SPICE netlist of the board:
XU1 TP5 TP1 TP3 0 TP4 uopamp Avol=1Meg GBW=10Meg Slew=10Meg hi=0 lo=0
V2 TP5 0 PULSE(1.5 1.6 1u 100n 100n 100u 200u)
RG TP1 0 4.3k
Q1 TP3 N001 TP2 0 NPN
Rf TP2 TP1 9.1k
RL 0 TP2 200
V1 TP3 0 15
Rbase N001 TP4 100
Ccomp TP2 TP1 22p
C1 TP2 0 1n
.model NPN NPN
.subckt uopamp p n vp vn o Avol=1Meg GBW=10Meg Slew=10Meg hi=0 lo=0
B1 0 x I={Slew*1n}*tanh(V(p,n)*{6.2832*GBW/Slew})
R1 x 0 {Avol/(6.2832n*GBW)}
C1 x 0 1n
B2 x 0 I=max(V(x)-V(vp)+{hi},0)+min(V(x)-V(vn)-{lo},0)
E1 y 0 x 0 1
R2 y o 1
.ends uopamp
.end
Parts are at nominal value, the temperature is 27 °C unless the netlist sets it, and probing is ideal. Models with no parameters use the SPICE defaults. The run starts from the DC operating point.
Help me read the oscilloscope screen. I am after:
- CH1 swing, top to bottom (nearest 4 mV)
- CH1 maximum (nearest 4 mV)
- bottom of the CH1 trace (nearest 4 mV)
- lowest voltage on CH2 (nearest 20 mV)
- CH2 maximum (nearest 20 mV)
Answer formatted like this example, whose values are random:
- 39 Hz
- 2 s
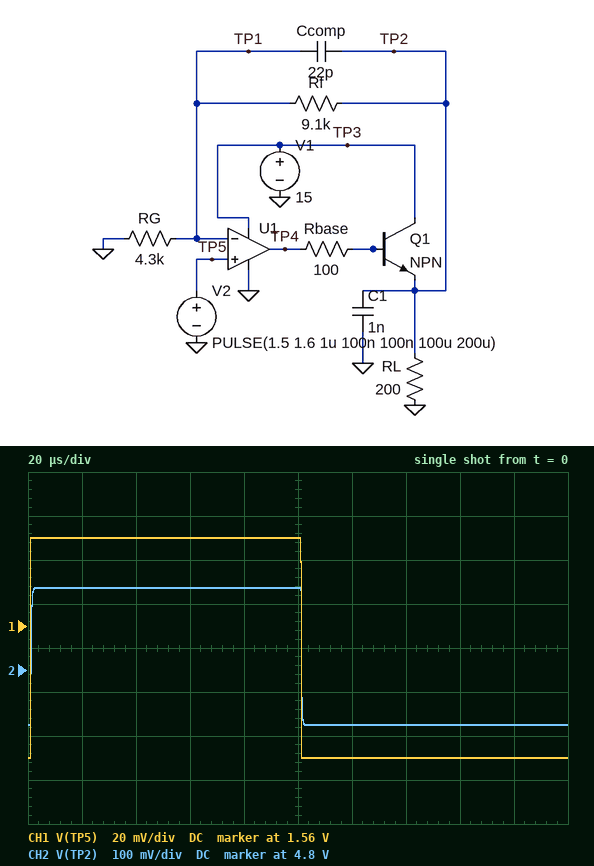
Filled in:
- 100 mV
- 1.600 V
- 1.500 V
- 4.68 V
- 4.98 V
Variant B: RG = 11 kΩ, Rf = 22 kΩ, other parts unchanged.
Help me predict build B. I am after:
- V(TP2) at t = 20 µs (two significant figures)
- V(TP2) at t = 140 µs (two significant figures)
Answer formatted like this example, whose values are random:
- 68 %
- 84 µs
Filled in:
- 4.8 V
- 4.5 V
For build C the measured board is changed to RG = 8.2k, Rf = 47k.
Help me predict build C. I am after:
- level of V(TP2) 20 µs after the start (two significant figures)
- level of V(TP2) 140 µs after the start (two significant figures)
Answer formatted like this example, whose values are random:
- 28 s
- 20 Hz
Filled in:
- 11 V
- 10 V
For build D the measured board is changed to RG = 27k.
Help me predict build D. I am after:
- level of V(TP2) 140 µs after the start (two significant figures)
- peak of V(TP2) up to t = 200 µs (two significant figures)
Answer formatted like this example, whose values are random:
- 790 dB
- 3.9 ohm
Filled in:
- 2.0 V
- 2.1 V
